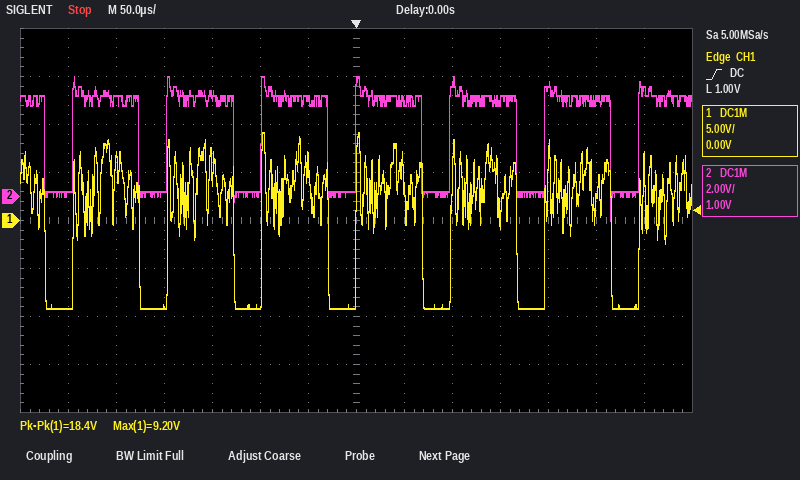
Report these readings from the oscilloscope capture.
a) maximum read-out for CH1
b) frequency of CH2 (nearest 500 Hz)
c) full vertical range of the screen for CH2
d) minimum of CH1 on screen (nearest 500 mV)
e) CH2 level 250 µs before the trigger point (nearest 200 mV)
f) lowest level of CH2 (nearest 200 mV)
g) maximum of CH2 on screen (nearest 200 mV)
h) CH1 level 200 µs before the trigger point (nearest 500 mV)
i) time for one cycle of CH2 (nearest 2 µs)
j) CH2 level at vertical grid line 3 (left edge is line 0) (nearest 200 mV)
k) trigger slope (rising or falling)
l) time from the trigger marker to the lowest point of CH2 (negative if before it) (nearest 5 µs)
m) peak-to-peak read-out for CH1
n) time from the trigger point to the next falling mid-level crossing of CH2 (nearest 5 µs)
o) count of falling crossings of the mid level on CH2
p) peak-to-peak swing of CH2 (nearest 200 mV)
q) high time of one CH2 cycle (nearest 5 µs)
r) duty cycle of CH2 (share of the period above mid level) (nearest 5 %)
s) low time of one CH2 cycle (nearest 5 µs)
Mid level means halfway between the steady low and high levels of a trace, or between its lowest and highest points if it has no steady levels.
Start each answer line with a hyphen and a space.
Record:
- 9.20 V
- 10.0 kHz
- 16 V
- -9.0 V
- 4.2 V
- -1.0 V
- 5.0 V
- -9.0 V
- 98 µs
- 200 mV
- rising
- +265 µs
- 18.4 V
- 70 µs
- 7
- 6.0 V
- 70 µs
- 70 %
- 30 µs
